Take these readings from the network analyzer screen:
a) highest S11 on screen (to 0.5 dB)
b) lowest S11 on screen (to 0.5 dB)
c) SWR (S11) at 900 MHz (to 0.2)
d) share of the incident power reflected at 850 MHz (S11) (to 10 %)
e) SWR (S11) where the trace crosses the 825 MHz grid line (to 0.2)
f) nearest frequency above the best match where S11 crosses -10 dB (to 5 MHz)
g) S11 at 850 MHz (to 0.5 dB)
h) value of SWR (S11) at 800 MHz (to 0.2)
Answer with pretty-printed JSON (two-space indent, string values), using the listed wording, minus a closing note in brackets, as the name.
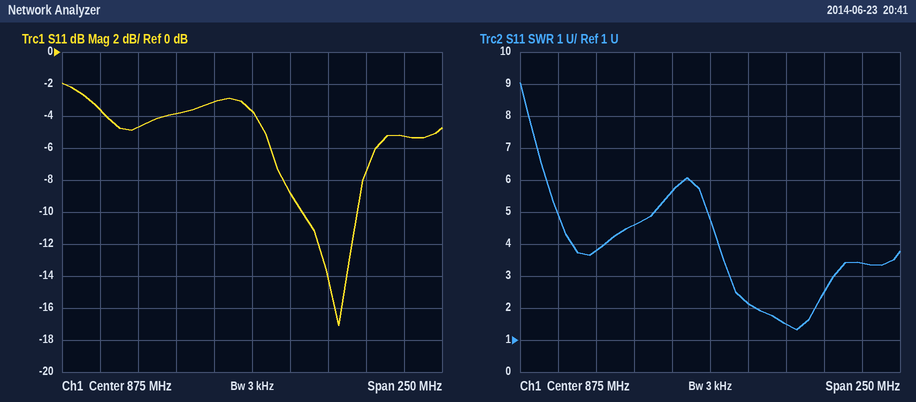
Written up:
{
  "highest S11 on screen": "-2.0 dB",
  "lowest S11 on screen": "-17.0 dB",
  "SWR (S11) at 900 MHz": "2.2",
  "share of the incident power reflected at 850 MHz (S11)": "50 %",
  "SWR (S11) where the trace crosses the 825 MHz grid line": "4.6",
  "nearest frequency above the best match where S11 crosses -10 dB": "945 MHz",
  "S11 at 850 MHz": "-3.0 dB",
  "value of SWR (S11) at 800 MHz": "3.8"
}
